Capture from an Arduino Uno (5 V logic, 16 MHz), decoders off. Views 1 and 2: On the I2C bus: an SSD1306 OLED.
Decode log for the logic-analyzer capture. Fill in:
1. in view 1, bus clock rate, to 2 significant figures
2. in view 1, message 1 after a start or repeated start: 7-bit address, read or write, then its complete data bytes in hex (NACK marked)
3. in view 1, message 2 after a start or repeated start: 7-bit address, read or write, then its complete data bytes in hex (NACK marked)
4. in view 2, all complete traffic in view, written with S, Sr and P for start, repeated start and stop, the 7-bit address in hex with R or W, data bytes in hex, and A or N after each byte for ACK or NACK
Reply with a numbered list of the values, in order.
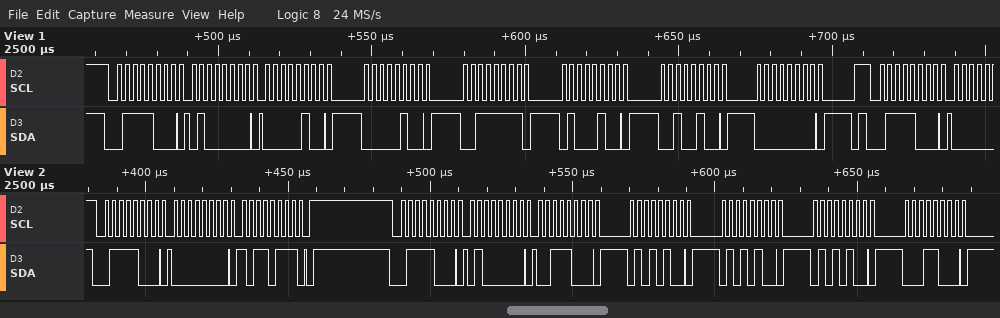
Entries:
1. 400 kHz
2. 0x3C write: 40 04 04 3F 44 24 00
3. 0x3C write
4. S 3CW A 00 A B7 A P S 3CW A 40 A 38 A 54 A 54 A 54 A 18 A
